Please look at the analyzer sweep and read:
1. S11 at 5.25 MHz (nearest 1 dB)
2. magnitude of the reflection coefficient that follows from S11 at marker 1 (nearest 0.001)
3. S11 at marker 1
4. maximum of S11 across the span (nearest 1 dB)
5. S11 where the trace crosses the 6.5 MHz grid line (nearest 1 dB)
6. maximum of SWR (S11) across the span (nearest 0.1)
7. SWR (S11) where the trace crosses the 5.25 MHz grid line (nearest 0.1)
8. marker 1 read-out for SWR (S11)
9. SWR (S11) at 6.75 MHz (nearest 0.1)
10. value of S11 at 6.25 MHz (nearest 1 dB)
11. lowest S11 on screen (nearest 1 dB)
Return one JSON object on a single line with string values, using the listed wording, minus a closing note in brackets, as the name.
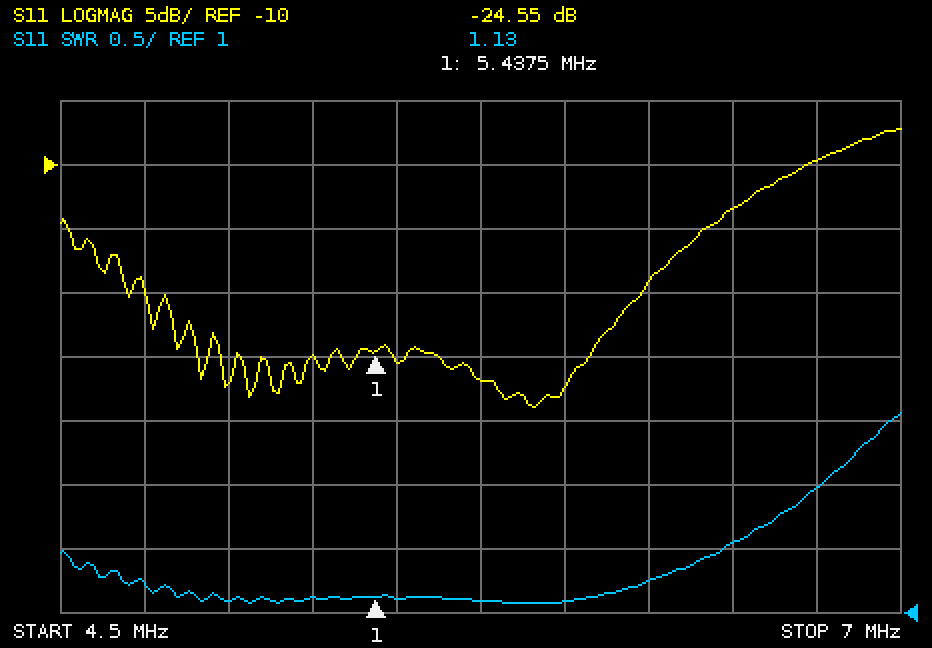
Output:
{"S11 at 5.25 MHz": "-25 dB", "magnitude of the reflection coefficient that follows from S11 at marker 1": "0.059", "S11 at marker 1": "-24.55 dB", "maximum of S11 across the span": "-7 dB", "S11 where the trace crosses the 6.5 MHz grid line": "-13 dB", "maximum of SWR (S11) across the span": "2.6", "SWR (S11) where the trace crosses the 5.25 MHz grid line": "1.1", "marker 1 read-out for SWR": "1.13", "SWR (S11) at 6.75 MHz": "2.0", "value of S11 at 6.25 MHz": "-19 dB", "lowest S11 on screen": "-29 dB"}
